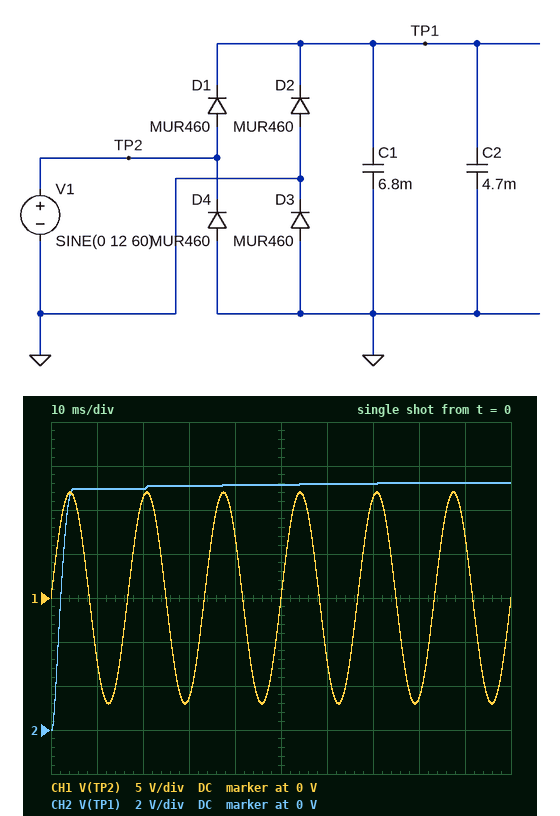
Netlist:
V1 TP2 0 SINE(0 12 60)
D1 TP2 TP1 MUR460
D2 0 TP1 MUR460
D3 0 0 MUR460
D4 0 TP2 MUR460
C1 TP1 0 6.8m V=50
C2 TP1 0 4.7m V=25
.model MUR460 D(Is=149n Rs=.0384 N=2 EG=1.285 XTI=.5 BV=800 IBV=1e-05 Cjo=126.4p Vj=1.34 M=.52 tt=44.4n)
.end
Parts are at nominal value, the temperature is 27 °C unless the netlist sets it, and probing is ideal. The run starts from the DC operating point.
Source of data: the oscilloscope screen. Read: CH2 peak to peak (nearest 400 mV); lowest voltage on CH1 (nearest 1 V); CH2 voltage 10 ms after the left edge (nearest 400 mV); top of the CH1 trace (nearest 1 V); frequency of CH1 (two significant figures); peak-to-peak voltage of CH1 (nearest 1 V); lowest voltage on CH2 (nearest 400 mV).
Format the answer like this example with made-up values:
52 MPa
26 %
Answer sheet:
11.2 V
-12 V
10.8 V
12 V
60 Hz
24 V
0 V
